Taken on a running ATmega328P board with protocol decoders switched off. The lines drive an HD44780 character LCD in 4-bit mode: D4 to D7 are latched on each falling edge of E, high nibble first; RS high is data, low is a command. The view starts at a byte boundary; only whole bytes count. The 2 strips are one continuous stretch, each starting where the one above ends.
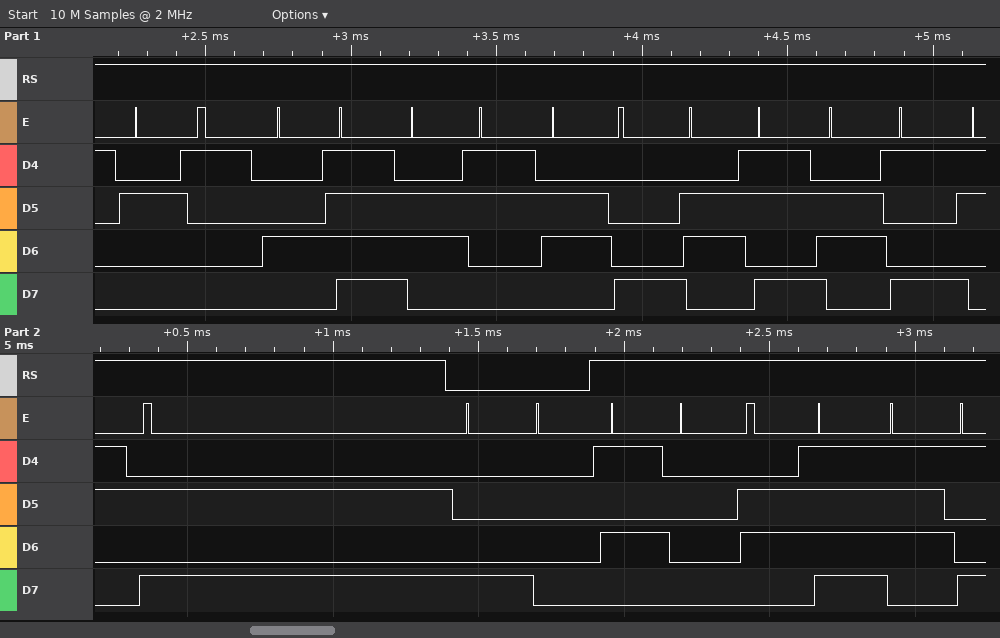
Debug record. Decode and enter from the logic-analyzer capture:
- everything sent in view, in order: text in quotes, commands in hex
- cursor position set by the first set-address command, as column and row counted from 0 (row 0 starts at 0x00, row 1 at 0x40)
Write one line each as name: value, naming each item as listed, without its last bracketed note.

everything sent in view, in order: text in quotes, commands in hex: "!Ochki:" 0x80 "Poy"
cursor position set by the first set-address command, as column and row counted from 0: column 0, row 0
